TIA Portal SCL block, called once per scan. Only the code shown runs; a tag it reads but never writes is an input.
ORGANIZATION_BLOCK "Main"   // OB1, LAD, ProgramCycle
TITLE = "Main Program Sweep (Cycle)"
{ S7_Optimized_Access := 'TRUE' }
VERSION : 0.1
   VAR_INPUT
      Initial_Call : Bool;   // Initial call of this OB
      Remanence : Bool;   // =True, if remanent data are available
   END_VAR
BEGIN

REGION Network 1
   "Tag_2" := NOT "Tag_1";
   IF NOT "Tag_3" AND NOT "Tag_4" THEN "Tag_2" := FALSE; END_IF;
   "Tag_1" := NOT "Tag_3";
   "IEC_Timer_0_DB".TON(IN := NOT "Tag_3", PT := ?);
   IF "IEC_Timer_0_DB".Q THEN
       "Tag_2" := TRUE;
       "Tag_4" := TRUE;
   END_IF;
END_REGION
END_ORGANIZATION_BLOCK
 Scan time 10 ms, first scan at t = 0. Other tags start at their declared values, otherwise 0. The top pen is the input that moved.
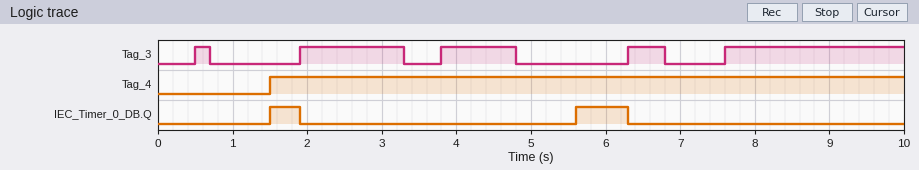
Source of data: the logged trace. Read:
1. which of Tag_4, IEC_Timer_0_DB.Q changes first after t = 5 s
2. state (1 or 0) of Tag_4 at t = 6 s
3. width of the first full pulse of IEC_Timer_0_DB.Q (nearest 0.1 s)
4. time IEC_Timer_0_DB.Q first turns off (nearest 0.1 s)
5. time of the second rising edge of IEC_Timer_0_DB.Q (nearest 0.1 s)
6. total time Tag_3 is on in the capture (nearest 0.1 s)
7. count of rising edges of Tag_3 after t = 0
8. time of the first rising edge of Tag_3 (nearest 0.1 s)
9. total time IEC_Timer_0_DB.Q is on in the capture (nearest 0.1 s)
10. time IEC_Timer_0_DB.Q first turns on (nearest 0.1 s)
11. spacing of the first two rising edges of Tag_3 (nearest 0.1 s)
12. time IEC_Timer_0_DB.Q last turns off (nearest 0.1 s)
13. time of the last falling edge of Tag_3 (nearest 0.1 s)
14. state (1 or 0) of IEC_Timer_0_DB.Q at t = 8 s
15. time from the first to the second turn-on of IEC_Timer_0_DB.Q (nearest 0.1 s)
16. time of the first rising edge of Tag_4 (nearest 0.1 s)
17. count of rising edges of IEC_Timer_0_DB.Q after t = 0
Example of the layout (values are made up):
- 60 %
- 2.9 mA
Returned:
- IEC_Timer_0_DB.Q
- 1
- 0.4 s
- 1.9 s
- 5.6 s
- 5.5 s
- 5
- 0.5 s
- 1.1 s
- 1.5 s
- 1.4 s
- 6.3 s
- 6.8 s
- 0
- 4.1 s
- 1.5 s
- 2
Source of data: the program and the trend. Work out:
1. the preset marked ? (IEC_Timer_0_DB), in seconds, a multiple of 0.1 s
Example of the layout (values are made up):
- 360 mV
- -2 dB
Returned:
- 0.8 s
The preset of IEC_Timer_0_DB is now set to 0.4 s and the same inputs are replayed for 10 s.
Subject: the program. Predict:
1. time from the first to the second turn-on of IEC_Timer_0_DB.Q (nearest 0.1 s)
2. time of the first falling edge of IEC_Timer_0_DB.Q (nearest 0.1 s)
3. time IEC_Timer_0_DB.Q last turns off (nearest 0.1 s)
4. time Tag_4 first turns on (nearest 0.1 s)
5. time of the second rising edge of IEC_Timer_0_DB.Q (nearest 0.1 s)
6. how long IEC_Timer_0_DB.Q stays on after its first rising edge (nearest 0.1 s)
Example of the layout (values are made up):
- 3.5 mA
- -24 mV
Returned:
- 0.7 s
- 0.5 s
- 7.6 s
- 0.4 s
- 1.1 s
- 0.1 s
